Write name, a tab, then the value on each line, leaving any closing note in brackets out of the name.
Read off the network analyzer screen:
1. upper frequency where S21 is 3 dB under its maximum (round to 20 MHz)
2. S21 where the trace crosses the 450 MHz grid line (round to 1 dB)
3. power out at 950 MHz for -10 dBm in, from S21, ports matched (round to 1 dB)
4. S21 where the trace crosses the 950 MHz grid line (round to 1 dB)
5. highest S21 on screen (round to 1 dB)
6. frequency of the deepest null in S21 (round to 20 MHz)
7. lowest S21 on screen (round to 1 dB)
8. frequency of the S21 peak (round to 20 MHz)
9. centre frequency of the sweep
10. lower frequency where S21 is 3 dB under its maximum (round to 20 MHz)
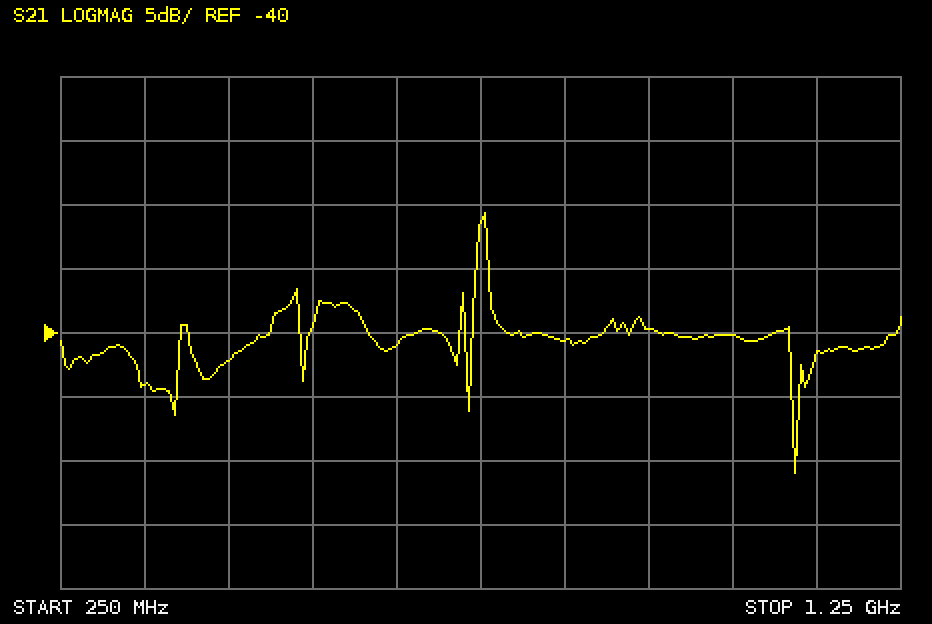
upper frequency where S21 is 3 dB under its maximum	760 MHz
S21 where the trace crosses the 450 MHz grid line	-42 dB
power out at 950 MHz for -10 dBm in, from S21, ports matched	-50 dBm
S21 where the trace crosses the 950 MHz grid line	-40 dB
highest S21 on screen	-31 dB
frequency of the deepest null in S21	1.12 GHz
lowest S21 on screen	-51 dB
frequency of the S21 peak	760 MHz
centre frequency of the sweep	750 MHz
lower frequency where S21 is 3 dB under its maximum	740 MHz
